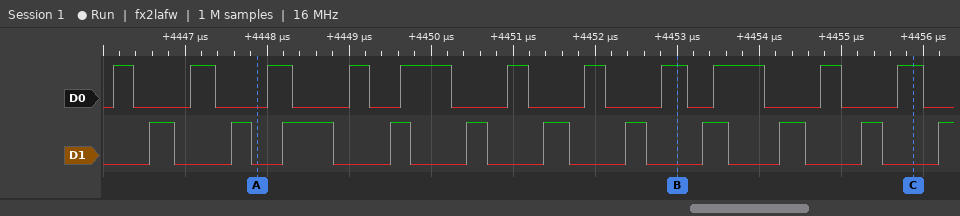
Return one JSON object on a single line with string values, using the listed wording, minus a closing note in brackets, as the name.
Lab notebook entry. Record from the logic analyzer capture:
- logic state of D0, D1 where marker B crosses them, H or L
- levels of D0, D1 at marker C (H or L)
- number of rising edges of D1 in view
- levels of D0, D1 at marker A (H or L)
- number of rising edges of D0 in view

{"logic state of D0, D1 where marker B crosses them, H or L": "D0=H, D1=L", "levels of D0, D1 at marker C": "D0=H, D1=L", "number of rising edges of D1 in view": "11", "levels of D0, D1 at marker A": "D0=L, D1=L", "number of rising edges of D0 in view": "11"}
